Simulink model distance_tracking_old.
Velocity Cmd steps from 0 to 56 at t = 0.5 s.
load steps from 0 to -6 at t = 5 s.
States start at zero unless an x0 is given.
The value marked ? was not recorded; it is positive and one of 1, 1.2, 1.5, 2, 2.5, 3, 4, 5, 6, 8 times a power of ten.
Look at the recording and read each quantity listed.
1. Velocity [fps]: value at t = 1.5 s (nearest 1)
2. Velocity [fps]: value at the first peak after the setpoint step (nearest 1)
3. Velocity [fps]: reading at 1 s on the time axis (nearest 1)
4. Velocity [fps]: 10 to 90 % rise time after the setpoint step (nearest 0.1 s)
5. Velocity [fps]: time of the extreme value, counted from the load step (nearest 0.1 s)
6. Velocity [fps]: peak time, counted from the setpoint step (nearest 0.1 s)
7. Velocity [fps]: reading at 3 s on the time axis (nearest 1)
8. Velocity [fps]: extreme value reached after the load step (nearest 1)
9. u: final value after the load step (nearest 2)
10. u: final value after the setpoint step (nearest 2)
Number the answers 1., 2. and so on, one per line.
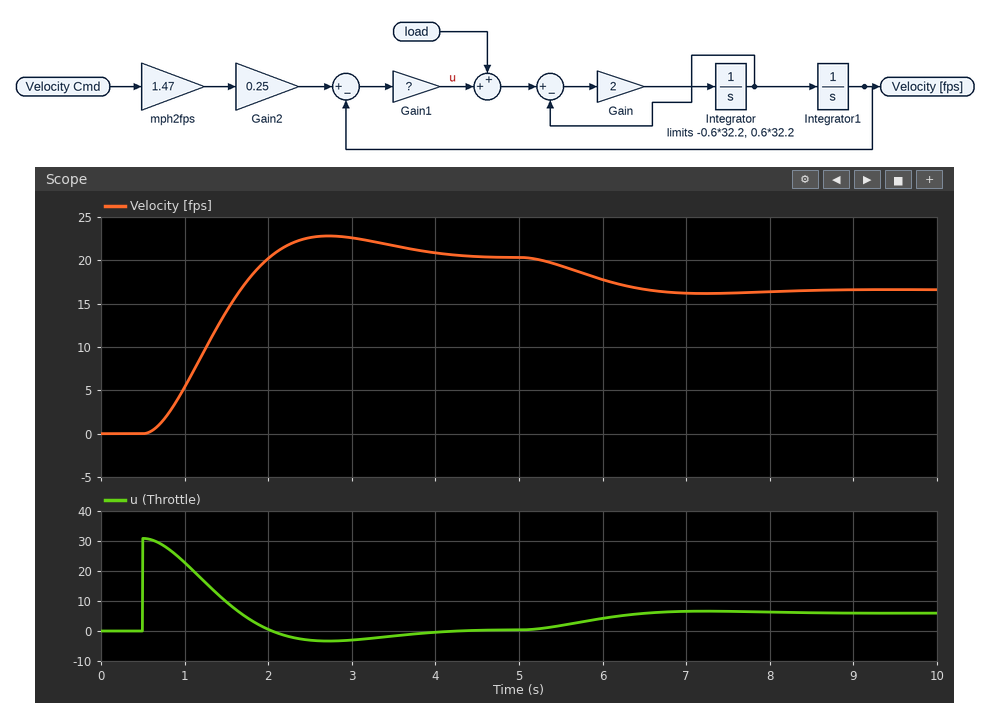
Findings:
1. 14
2. 23
3. 5
4. 1.0 s
5. 2.2 s
6. 2.2 s
7. 23
8. 16
9. 6
10. 0
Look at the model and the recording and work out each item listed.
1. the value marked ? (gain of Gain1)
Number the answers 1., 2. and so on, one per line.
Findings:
1. 1.5
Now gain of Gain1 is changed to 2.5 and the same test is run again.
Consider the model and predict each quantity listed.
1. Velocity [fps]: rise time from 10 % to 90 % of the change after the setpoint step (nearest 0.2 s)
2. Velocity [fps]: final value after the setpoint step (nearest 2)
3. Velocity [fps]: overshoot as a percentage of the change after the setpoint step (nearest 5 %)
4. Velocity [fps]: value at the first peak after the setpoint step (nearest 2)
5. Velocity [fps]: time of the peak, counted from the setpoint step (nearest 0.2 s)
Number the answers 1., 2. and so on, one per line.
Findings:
1. 0.8 s
2. 20
3. 15 %
4. 24
5. 1.8 s
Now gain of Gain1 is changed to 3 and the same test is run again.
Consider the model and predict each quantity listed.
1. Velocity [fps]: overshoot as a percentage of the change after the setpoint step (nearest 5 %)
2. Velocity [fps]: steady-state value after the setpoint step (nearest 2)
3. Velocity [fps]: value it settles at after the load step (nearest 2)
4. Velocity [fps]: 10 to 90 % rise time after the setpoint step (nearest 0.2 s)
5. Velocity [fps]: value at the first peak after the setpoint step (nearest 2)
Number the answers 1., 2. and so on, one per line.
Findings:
1. 15 %
2. 20
3. 18
4. 0.8 s
5. 24
